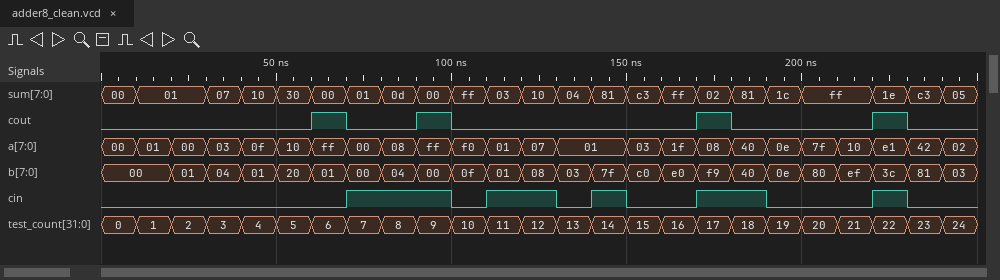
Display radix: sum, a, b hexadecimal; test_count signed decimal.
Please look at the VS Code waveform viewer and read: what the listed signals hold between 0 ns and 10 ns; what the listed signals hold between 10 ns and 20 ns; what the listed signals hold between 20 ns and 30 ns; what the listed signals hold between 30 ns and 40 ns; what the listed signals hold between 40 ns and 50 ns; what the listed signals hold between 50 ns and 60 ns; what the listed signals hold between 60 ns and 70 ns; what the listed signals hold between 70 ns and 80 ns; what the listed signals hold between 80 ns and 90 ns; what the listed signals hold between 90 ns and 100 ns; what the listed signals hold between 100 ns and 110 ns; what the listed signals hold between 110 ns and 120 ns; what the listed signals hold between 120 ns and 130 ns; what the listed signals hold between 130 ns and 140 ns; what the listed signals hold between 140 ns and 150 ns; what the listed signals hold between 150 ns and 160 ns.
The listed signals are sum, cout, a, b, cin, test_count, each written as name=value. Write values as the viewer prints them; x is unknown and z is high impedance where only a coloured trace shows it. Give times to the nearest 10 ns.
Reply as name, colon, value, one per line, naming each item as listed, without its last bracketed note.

what the listed signals hold between 0 ns and 10 ns: sum=00, cout=0, a=00, b=00, cin=0, test_count=0
what the listed signals hold between 10 ns and 20 ns: sum=01, cout=0, a=01, b=00, cin=0, test_count=1
what the listed signals hold between 20 ns and 30 ns: sum=01, cout=0, a=00, b=01, cin=0, test_count=2
what the listed signals hold between 30 ns and 40 ns: sum=07, cout=0, a=03, b=04, cin=0, test_count=3
what the listed signals hold between 40 ns and 50 ns: sum=10, cout=0, a=0f, b=01, cin=0, test_count=4
what the listed signals hold between 50 ns and 60 ns: sum=30, cout=0, a=10, b=20, cin=0, test_count=5
what the listed signals hold between 60 ns and 70 ns: sum=00, cout=1, a=ff, b=01, cin=0, test_count=6
what the listed signals hold between 70 ns and 80 ns: sum=01, cout=0, a=00, b=00, cin=1, test_count=7
what the listed signals hold between 80 ns and 90 ns: sum=0d, cout=0, a=08, b=04, cin=1, test_count=8
what the listed signals hold between 90 ns and 100 ns: sum=00, cout=1, a=ff, b=00, cin=1, test_count=9
what the listed signals hold between 100 ns and 110 ns: sum=ff, cout=0, a=f0, b=0f, cin=0, test_count=10
what the listed signals hold between 110 ns and 120 ns: sum=03, cout=0, a=01, b=01, cin=1, test_count=11
what the listed signals hold between 120 ns and 130 ns: sum=10, cout=0, a=07, b=08, cin=1, test_count=12
what the listed signals hold between 130 ns and 140 ns: sum=04, cout=0, a=01, b=03, cin=0, test_count=13
what the listed signals hold between 140 ns and 150 ns: sum=81, cout=0, a=01, b=7f, cin=1, test_count=14
what the listed signals hold between 150 ns and 160 ns: sum=c3, cout=0, a=03, b=c0, cin=0, test_count=15
